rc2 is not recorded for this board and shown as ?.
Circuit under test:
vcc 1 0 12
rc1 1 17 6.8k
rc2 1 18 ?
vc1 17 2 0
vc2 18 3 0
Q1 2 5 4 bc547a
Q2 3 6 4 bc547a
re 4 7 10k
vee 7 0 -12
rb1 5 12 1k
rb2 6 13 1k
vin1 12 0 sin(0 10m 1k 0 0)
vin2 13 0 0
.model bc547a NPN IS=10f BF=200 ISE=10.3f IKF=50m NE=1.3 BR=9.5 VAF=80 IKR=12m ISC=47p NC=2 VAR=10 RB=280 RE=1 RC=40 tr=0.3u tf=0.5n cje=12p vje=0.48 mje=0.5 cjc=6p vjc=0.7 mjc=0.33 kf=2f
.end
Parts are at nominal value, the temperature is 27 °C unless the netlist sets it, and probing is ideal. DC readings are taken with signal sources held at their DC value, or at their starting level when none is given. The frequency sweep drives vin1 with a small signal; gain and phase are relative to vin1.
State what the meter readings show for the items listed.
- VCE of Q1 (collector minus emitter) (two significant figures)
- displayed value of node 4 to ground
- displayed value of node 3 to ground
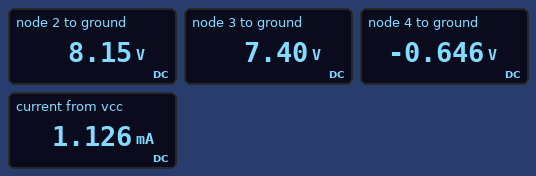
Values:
8.8 V
-0.646 V
7.40 V
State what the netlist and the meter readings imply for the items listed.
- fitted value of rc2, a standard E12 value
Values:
8.2 kΩ
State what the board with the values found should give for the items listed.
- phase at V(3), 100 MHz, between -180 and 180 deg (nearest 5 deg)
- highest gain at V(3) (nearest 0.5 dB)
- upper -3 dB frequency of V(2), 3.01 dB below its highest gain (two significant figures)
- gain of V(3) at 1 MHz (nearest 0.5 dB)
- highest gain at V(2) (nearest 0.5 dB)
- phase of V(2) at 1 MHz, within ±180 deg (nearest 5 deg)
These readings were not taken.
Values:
-10 deg
36.5 dB
330 kHz
26.5 dB
35.0 dB
110 deg
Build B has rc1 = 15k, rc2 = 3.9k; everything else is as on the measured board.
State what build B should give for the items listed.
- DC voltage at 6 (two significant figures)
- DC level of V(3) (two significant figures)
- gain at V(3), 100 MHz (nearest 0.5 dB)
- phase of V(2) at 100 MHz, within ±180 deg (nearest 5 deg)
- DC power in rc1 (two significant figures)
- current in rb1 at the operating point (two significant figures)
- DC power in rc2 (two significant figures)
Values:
-4.7 mV
9.7 V
-11.0 dB
10 deg
4.4 mW
4.7 µA
1.3 mW
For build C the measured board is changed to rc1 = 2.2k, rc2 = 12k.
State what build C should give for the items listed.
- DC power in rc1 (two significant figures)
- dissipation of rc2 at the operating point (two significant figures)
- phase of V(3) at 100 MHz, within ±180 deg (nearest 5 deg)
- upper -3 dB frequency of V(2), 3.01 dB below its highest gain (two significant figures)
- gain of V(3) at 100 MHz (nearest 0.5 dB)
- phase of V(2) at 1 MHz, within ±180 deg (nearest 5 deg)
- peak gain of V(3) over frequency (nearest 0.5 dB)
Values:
740 µW
3.6 mW
-15 deg
320 kHz
-11.5 dB
115 deg
40.0 dB
